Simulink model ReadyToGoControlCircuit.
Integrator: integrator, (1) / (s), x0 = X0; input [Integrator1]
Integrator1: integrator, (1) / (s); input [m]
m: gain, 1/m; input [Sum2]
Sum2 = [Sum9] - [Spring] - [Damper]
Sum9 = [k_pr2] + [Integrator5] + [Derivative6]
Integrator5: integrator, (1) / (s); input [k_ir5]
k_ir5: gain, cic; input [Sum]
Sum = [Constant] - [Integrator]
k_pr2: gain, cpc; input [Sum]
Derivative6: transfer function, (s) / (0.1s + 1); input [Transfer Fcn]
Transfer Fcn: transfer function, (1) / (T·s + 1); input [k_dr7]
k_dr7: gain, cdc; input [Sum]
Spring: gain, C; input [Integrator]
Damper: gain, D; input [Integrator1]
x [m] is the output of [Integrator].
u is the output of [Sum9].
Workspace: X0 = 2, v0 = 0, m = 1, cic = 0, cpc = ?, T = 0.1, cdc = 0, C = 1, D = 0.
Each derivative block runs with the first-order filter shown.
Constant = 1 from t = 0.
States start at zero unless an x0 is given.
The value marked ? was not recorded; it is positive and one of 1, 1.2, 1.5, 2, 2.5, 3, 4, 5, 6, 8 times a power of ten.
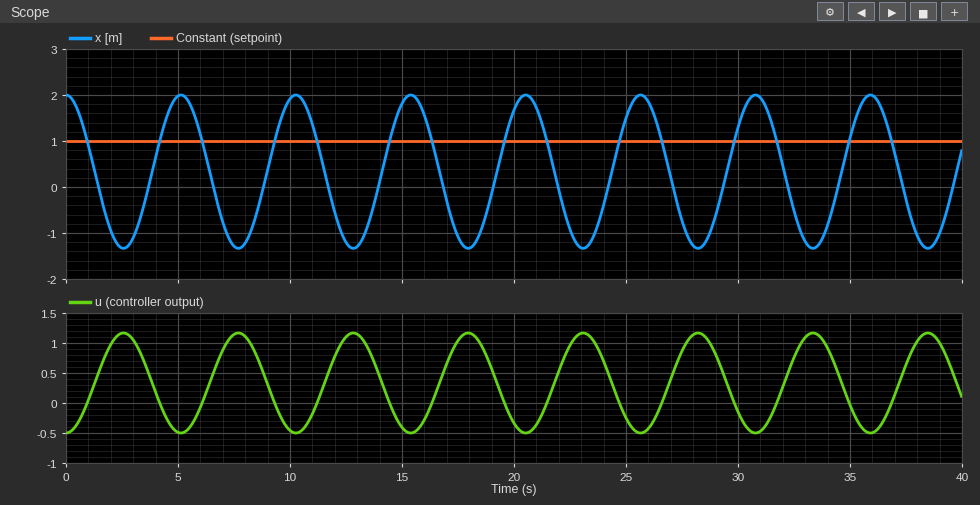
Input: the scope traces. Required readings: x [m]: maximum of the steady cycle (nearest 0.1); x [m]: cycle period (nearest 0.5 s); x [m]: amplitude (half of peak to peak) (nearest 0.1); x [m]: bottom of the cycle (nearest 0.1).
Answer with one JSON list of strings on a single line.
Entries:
["2.0", "5.0 s", "1.7", "-1.3"]
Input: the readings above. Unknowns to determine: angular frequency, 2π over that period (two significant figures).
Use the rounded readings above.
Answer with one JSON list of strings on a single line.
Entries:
["1.3 rad/s"]
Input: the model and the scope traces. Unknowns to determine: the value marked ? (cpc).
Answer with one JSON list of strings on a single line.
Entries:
["0.5"]
